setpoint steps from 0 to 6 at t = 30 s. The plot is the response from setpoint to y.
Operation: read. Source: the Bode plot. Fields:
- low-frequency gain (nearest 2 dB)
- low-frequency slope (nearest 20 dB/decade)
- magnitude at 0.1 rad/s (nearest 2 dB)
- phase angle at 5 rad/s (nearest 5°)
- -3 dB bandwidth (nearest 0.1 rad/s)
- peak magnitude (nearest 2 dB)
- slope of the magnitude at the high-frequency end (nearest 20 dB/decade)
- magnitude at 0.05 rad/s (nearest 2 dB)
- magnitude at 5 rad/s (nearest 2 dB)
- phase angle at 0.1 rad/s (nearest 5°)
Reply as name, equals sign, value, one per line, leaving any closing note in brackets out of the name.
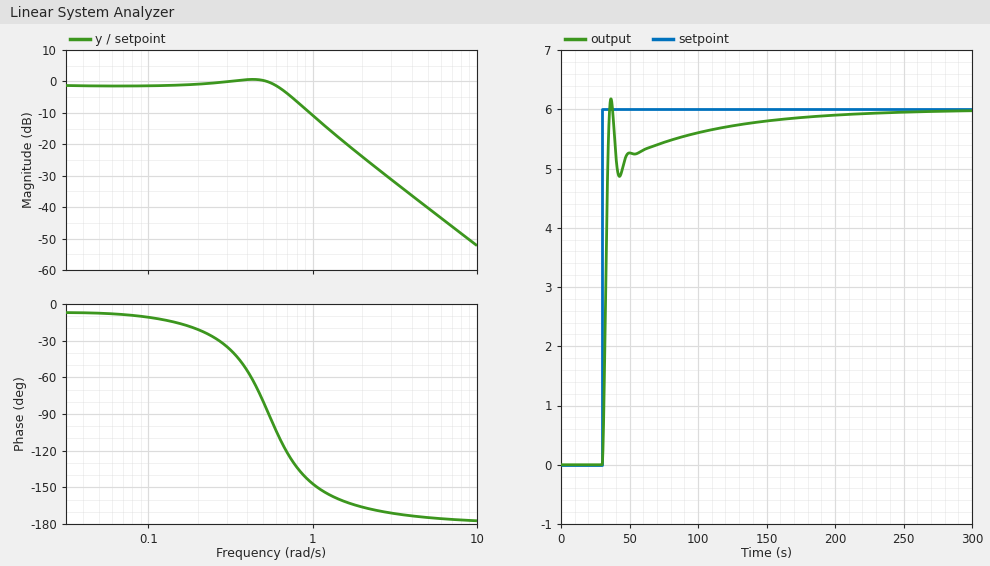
low-frequency gain = -2 dB
low-frequency slope = 0 dB/decade
magnitude at 0.1 rad/s = -2 dB
phase angle at 5 rad/s = -175°
-3 dB bandwidth = 0.7 rad/s
peak magnitude = 0 dB
slope of the magnitude at the high-frequency end = -40 dB/decade
magnitude at 0.05 rad/s = -2 dB
magnitude at 5 rad/s = -40 dB
phase angle at 0.1 rad/s = -10°
